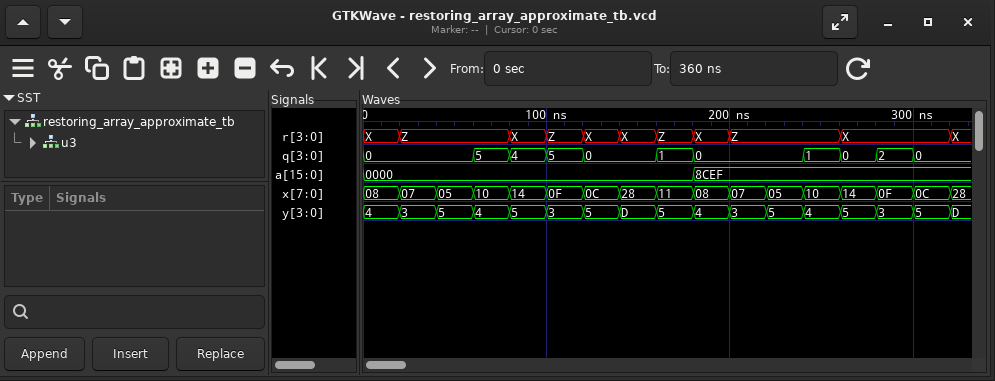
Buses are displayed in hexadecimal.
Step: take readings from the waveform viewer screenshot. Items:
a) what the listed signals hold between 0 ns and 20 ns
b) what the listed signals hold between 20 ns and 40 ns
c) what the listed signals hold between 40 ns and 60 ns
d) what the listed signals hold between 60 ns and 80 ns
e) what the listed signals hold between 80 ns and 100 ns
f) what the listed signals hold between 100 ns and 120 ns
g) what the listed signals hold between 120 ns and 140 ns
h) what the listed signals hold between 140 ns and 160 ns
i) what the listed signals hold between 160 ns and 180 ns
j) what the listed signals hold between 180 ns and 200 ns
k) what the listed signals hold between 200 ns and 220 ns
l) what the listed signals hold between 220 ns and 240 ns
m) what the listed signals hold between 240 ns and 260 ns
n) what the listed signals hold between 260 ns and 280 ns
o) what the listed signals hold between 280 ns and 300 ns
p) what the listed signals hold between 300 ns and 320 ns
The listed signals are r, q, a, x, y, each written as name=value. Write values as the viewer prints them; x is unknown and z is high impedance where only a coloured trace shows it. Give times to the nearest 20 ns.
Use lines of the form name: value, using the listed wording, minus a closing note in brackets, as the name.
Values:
what the listed signals hold between 0 ns and 20 ns: r=X, q=0, a=0000, x=08, y=4
what the listed signals hold between 20 ns and 40 ns: r=Z, q=0, a=0000, x=07, y=3
what the listed signals hold between 40 ns and 60 ns: r=Z, q=0, a=0000, x=05, y=5
what the listed signals hold between 60 ns and 80 ns: r=Z, q=5, a=0000, x=10, y=4
what the listed signals hold between 80 ns and 100 ns: r=X, q=4, a=0000, x=14, y=5
what the listed signals hold between 100 ns and 120 ns: r=Z, q=5, a=0000, x=0F, y=3
what the listed signals hold between 120 ns and 140 ns: r=X, q=0, a=0000, x=0C, y=5
what the listed signals hold between 140 ns and 160 ns: r=X, q=0, a=0000, x=28, y=D
what the listed signals hold between 160 ns and 180 ns: r=Z, q=1, a=0000, x=11, y=5
what the listed signals hold between 180 ns and 200 ns: r=X, q=0, a=8CEF, x=08, y=4
what the listed signals hold between 200 ns and 220 ns: r=Z, q=0, a=8CEF, x=07, y=3
what the listed signals hold between 220 ns and 240 ns: r=Z, q=0, a=8CEF, x=05, y=5
what the listed signals hold between 240 ns and 260 ns: r=Z, q=1, a=8CEF, x=10, y=4
what the listed signals hold between 260 ns and 280 ns: r=X, q=0, a=8CEF, x=14, y=5
what the listed signals hold between 280 ns and 300 ns: r=X, q=2, a=8CEF, x=0F, y=3
what the listed signals hold between 300 ns and 320 ns: r=X, q=0, a=8CEF, x=0C, y=5
